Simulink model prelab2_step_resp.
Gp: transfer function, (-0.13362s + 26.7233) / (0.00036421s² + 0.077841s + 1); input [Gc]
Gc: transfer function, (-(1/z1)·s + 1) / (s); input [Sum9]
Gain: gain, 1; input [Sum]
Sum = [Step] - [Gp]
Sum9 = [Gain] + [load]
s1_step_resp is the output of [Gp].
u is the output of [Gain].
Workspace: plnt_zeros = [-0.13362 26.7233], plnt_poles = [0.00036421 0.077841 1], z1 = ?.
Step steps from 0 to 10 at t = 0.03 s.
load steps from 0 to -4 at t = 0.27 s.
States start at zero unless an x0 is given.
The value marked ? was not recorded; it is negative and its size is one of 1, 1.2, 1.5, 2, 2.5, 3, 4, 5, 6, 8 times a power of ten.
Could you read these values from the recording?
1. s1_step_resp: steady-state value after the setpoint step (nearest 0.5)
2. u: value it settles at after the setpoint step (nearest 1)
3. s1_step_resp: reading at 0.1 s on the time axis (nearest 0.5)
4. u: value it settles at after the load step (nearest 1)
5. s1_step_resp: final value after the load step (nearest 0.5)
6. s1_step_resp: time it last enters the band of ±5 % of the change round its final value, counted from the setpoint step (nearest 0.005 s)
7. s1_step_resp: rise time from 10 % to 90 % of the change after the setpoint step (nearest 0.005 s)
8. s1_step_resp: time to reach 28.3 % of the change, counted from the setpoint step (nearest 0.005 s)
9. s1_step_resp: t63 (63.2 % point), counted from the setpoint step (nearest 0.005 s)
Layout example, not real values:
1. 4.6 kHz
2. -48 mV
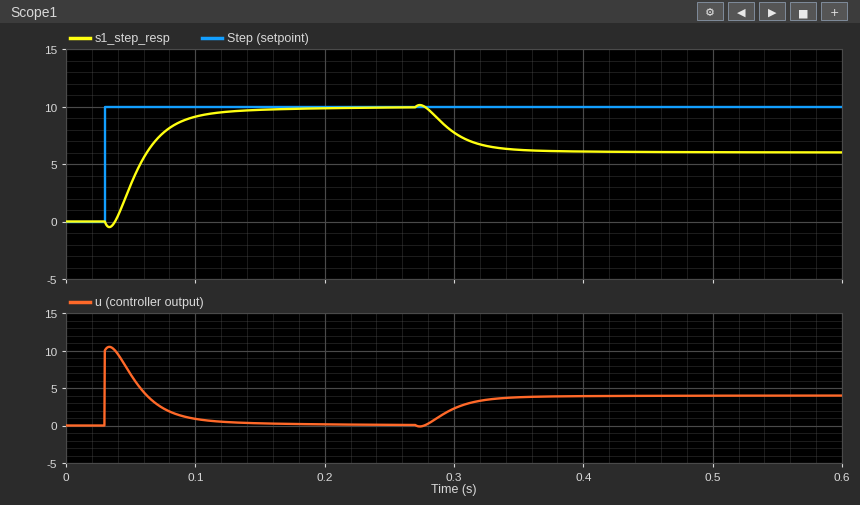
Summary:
1. 10.0
2. 0
3. 9.0
4. 4
5. 6.0
6. 0.090 s
7. 0.055 s
8. 0.020 s
9. 0.035 s
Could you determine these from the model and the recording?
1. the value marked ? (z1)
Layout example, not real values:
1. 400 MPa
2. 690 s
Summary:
1. -12
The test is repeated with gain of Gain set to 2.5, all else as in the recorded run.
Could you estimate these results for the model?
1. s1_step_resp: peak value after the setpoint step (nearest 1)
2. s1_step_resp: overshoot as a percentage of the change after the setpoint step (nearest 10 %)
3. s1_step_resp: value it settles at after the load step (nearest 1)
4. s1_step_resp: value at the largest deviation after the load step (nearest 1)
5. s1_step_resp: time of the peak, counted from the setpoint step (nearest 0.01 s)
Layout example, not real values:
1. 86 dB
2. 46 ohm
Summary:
1. 12
2. 20 %
3. 8
4. 8
5. 0.03 s
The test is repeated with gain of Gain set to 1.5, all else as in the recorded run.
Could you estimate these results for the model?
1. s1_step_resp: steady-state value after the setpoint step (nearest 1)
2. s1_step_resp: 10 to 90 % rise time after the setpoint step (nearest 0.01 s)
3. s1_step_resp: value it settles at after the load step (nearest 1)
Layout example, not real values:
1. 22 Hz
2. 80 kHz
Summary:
1. 10
2. 0.03 s
3. 7
